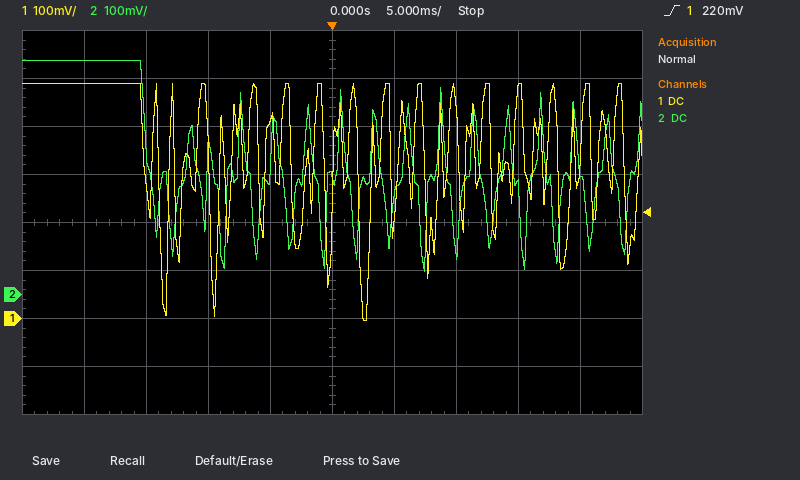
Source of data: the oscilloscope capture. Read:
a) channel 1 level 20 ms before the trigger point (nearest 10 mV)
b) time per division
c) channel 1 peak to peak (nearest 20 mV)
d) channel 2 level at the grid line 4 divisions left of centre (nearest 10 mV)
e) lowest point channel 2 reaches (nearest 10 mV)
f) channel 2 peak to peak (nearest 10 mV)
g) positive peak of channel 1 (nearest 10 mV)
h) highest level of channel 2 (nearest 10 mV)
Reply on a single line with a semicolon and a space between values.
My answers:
490 mV; 5 ms; 500 mV; 490 mV; 50 mV; 440 mV; 490 mV; 490 mV
